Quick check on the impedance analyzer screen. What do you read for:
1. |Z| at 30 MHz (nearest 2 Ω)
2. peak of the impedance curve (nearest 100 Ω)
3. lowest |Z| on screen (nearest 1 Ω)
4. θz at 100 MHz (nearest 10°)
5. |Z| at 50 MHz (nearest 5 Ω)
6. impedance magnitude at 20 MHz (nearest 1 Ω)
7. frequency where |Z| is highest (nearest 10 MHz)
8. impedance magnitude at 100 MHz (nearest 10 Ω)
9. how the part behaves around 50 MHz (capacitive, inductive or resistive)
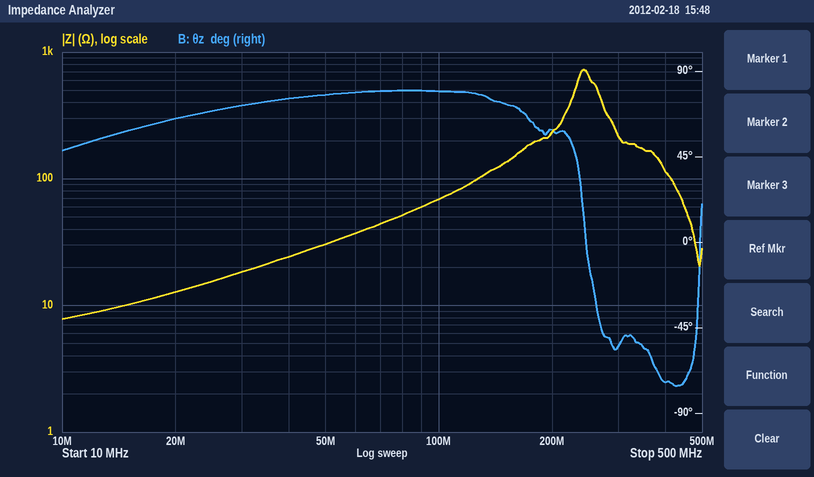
18 Ω
700 Ω
8 Ω
80°
30 Ω
13 Ω
240 MHz
70 Ω
inductive
